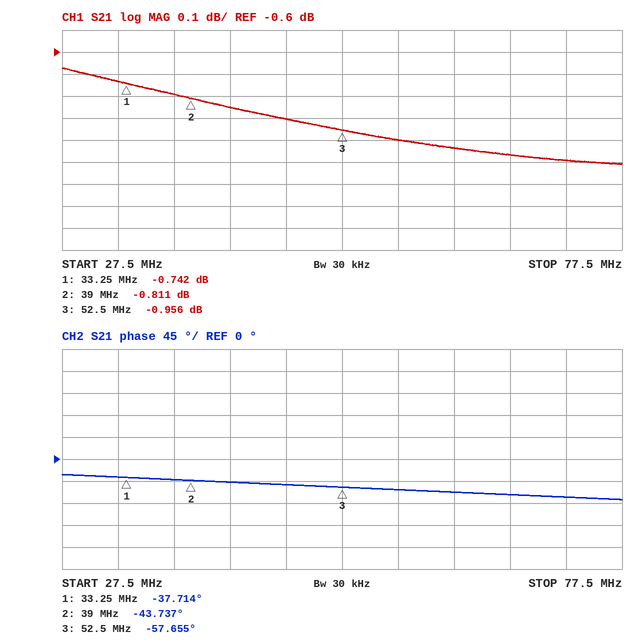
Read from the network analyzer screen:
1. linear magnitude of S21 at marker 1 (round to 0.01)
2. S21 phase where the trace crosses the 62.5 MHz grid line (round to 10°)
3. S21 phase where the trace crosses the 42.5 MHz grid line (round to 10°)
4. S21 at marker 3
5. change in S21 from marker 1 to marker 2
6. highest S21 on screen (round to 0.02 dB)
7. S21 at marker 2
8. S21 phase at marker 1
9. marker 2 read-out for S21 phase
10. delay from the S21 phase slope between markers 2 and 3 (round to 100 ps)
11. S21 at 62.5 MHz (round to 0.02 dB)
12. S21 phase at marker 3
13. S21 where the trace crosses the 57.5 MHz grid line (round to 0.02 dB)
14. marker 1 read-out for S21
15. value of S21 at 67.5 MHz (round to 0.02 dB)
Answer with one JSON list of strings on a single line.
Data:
["0.92", "-70°", "-50°", "-0.956 dB", "-0.069 dB", "-0.68 dB", "-0.811 dB", "-37.714°", "-43.737°", "2.9 ns", "-1.04 dB", "-57.655°", "-1.00 dB", "-0.742 dB", "-1.06 dB"]
